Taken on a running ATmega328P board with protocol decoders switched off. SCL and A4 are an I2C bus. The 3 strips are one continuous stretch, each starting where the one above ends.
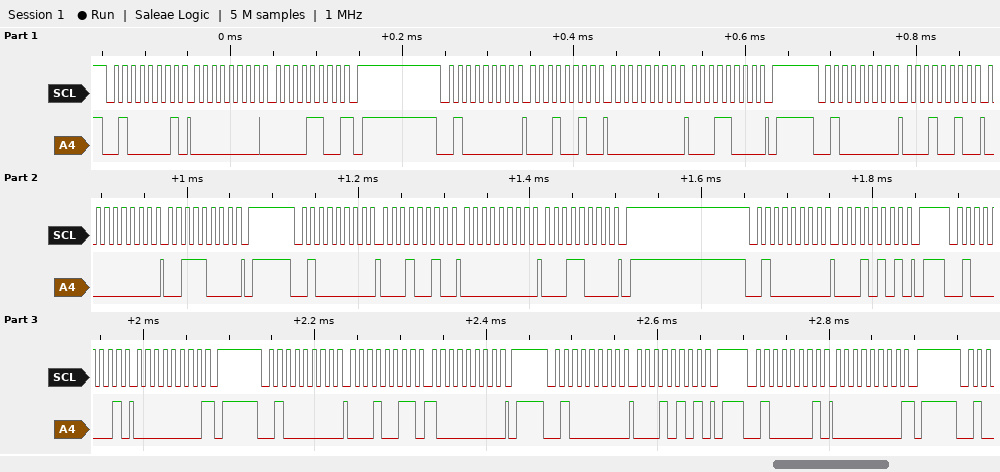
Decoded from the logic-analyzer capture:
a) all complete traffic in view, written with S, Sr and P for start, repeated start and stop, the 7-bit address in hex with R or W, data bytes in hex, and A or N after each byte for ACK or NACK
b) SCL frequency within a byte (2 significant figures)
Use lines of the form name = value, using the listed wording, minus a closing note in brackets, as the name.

all complete traffic in view, written with S, Sr and P for start, repeated start and stop, the 7-bit address in hex with R or W, data bytes in hex, and A or N after each byte for ACK or NACK = S 20R A 00 A 0C N P S 20W A 12 A 00 A 18 A P S 20W A 12 A 00 A 38 A P S 20W A 12 A 00 A 18 A P S 20W A 15 A P S 20R A 00 N P S 20W A 13 A 80 A P S 20W A 15 A P S 20R A 00 N P
SCL frequency within a byte = 100 kHz
